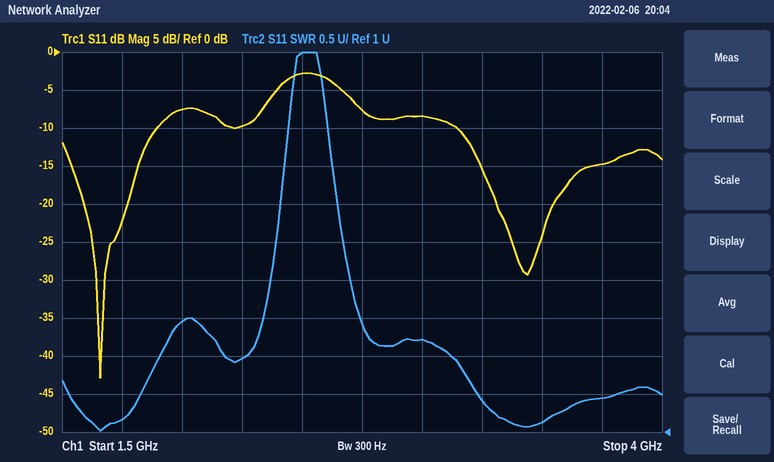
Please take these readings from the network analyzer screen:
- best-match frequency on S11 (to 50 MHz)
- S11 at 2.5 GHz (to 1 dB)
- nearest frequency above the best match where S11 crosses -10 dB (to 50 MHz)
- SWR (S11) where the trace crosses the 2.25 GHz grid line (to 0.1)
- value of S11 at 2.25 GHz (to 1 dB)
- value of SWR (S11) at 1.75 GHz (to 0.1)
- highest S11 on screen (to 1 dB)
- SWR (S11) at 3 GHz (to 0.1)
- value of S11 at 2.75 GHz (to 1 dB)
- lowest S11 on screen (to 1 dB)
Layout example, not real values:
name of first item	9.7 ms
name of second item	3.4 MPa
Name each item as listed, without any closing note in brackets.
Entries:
best-match frequency on S11	1.65 GHz
S11 at 2.5 GHz	-3 dB
nearest frequency above the best match where S11 crosses -10 dB	1.90 GHz
SWR (S11) where the trace crosses the 2.25 GHz grid line	2.0
value of S11 at 2.25 GHz	-10 dB
value of SWR (S11) at 1.75 GHz	1.2
highest S11 on screen	-3 dB
SWR (S11) at 3 GHz	2.2
value of S11 at 2.75 GHz	-8 dB
lowest S11 on screen	-43 dB
